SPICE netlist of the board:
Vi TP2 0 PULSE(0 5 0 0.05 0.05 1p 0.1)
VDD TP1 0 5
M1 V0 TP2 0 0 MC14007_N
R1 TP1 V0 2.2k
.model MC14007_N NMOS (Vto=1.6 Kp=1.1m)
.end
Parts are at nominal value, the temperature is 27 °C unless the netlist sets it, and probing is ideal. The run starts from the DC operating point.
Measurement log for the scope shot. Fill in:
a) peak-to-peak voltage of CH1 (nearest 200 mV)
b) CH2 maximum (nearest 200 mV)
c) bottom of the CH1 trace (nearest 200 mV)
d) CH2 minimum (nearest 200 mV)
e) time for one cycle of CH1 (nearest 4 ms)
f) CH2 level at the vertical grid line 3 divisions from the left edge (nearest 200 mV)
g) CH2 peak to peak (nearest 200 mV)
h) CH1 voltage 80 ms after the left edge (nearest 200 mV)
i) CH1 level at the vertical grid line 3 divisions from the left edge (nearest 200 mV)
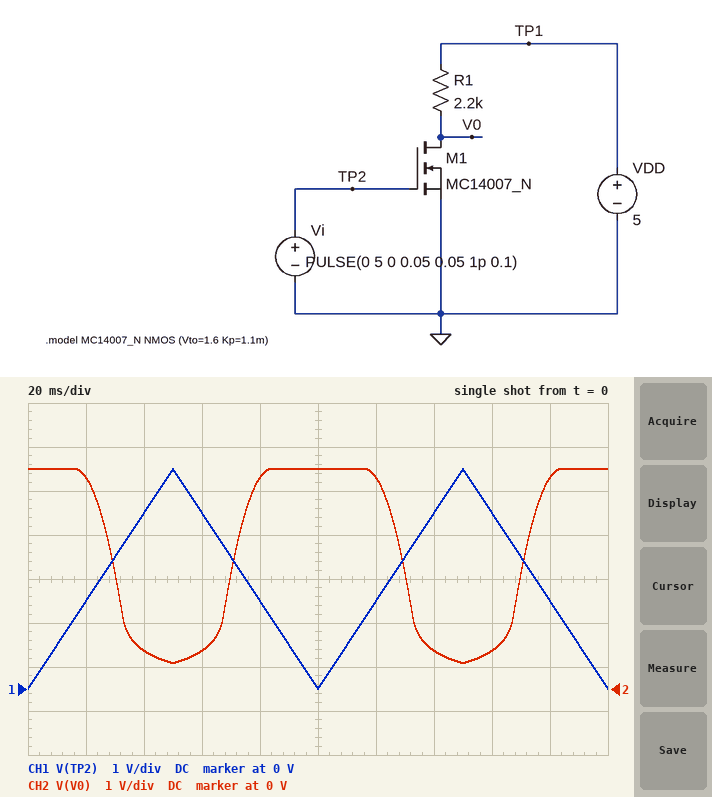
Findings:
5.0 V
5.0 V
0 V
600 mV
100 ms
800 mV
4.4 V
2.0 V
4.0 V
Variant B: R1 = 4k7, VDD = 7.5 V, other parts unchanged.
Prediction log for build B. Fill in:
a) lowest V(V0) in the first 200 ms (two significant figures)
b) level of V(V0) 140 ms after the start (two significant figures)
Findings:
430 mV
640 mV
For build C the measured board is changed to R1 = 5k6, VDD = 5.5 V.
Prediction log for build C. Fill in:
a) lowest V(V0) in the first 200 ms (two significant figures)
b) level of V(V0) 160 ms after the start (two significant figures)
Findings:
260 mV
380 mV
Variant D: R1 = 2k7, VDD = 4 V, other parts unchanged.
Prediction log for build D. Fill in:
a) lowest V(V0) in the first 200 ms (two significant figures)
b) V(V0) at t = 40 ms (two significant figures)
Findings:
380 mV
550 mV
